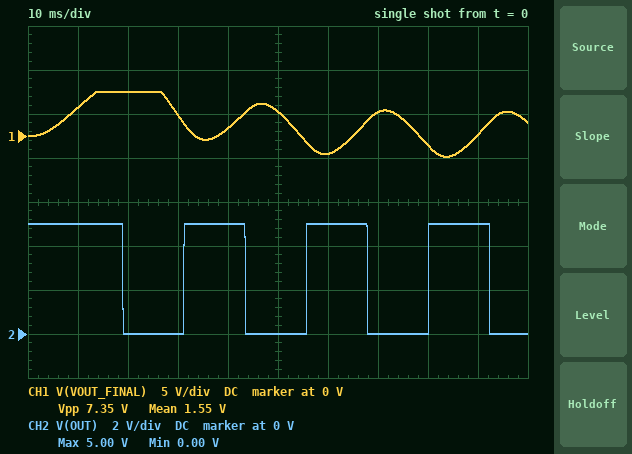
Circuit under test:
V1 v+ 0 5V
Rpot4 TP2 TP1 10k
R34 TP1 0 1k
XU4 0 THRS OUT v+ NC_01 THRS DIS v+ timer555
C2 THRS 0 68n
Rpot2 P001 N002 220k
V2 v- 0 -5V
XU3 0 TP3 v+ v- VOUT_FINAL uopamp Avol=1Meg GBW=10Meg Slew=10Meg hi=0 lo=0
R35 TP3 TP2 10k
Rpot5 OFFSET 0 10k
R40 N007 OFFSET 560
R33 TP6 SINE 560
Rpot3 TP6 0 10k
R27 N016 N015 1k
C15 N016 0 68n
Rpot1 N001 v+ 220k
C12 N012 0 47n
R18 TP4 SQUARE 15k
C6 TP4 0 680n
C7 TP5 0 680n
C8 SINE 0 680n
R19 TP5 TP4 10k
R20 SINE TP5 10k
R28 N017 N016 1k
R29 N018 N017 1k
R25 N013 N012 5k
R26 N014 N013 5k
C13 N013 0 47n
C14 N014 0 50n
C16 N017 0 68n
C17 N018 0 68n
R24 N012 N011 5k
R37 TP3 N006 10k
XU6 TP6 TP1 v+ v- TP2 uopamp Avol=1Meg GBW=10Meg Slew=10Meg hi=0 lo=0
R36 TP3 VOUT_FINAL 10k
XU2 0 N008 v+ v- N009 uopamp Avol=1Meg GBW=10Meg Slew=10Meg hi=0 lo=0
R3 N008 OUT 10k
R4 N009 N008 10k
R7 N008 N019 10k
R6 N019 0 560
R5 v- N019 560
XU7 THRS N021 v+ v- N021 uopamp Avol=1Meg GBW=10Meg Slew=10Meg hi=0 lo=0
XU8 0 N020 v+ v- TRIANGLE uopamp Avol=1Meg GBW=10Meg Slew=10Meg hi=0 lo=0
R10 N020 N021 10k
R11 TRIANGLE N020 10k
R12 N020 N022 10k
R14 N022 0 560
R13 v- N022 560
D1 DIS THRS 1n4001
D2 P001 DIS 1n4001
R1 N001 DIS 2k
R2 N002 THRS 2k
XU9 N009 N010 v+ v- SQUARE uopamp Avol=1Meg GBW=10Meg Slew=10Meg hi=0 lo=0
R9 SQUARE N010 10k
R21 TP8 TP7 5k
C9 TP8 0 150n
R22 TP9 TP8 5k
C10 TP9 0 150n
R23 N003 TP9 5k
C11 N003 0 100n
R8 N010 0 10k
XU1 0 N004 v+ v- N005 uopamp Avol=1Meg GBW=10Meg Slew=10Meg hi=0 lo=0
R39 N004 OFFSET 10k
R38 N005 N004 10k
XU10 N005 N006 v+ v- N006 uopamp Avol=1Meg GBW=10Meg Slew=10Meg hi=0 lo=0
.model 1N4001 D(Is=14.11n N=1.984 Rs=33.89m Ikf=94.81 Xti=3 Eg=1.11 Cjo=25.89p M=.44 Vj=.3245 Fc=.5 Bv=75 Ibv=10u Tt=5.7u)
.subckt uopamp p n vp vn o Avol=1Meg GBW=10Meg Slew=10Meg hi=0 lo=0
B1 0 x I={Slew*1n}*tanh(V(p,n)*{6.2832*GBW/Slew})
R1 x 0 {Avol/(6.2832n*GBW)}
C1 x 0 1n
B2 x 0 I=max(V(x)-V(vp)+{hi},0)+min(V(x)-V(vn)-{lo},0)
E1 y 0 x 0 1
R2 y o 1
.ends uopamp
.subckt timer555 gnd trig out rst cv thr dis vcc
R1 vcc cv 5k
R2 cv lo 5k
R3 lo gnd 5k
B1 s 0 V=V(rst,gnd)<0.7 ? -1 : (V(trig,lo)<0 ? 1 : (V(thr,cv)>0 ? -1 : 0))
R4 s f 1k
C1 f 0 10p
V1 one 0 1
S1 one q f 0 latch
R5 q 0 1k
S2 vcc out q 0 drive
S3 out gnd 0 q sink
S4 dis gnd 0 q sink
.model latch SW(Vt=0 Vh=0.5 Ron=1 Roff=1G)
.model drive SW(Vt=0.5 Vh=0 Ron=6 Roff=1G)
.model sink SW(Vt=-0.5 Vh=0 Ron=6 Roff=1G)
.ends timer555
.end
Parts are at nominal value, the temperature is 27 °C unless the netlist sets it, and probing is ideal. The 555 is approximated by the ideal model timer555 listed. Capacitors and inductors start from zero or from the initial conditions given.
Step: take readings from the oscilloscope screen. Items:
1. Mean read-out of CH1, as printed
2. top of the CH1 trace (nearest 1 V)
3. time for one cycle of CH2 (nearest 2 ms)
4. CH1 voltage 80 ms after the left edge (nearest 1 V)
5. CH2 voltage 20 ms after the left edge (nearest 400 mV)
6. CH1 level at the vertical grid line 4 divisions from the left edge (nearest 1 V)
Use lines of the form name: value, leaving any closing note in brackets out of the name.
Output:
Mean read-out of CH1, as printed: 1.55 V
top of the CH1 trace: 5 V
time for one cycle of CH2: 24 ms
CH1 voltage 80 ms after the left edge: -1 V
CH2 voltage 20 ms after the left edge: 0 V
CH1 level at the vertical grid line 4 divisions from the left edge: 1 V
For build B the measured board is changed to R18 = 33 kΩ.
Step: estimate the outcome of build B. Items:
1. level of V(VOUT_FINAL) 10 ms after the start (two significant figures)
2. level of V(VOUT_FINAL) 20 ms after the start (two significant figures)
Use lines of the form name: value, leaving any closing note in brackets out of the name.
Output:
level of V(VOUT_FINAL) 10 ms after the start: 1.7 V
level of V(VOUT_FINAL) 20 ms after the start: 4.2 V
